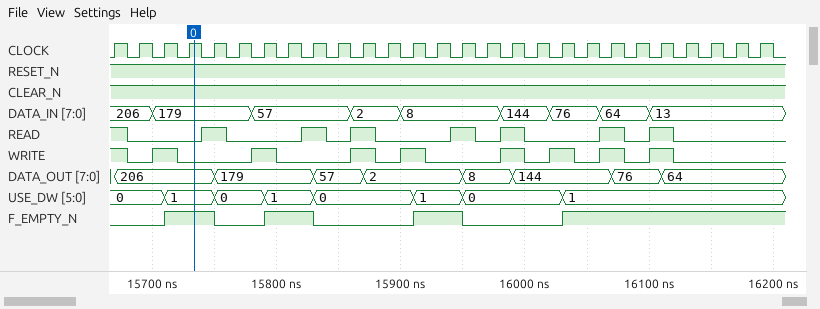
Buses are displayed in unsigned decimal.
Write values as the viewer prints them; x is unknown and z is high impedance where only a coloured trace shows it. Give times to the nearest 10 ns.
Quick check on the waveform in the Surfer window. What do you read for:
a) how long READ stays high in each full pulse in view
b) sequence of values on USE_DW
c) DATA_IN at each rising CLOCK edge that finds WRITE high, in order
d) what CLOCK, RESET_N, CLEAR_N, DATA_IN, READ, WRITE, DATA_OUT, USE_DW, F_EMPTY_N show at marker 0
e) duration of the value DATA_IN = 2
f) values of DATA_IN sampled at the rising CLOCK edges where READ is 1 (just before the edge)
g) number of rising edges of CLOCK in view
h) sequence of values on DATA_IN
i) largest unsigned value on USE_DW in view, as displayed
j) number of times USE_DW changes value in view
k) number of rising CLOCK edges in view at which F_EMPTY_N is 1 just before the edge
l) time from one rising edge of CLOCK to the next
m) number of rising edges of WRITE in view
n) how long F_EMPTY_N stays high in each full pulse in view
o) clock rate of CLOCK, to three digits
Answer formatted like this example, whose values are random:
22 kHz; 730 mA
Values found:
20 ns, 20 ns, 20 ns, 20 ns, 20 ns, 20 ns, 20 ns; 0, 1, 0, 1, 0, 1, 0, 1; 206, 179, 57, 2, 8, 144, 76, 64, 13; CLOCK=1, RESET_N=1, CLEAR_N=1, DATA_IN=179, READ=0, WRITE=0, DATA_OUT=206, USE_DW=1, F_EMPTY_N=1; 40 ns; 206, 179, 57, 2, 8, 144, 64, 13; 27; 206, 179, 57, 2, 8, 144, 76, 64, 13; 1; 7; 14; 20 ns; 8; 40 ns, 40 ns, 40 ns; 50.0 MHz
